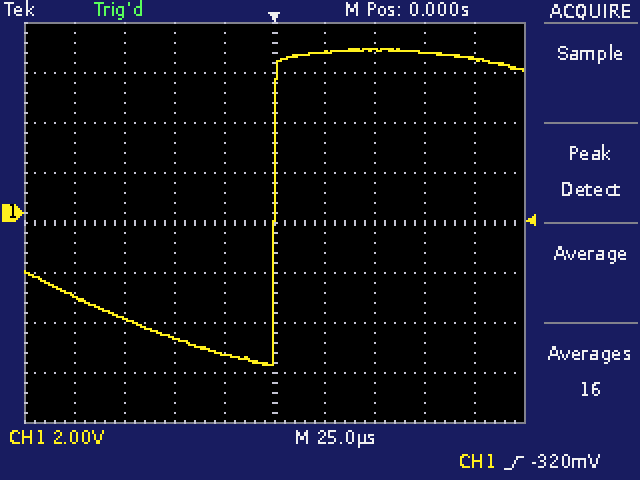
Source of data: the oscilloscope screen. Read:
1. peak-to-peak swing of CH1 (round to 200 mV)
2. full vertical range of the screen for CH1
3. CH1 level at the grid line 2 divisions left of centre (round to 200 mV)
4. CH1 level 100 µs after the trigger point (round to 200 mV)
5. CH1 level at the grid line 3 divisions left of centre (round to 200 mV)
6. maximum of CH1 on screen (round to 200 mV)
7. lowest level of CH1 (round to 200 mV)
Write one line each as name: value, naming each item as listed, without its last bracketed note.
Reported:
peak-to-peak swing of CH1: 12.6 V
full vertical range of the screen for CH1: 16 V
CH1 level at the grid line 2 divisions left of centre: -5.0 V
CH1 level 100 µs after the trigger point: 6.2 V
CH1 level at the grid line 3 divisions left of centre: -4.2 V
maximum of CH1 on screen: 6.6 V
lowest level of CH1: -6.0 V
